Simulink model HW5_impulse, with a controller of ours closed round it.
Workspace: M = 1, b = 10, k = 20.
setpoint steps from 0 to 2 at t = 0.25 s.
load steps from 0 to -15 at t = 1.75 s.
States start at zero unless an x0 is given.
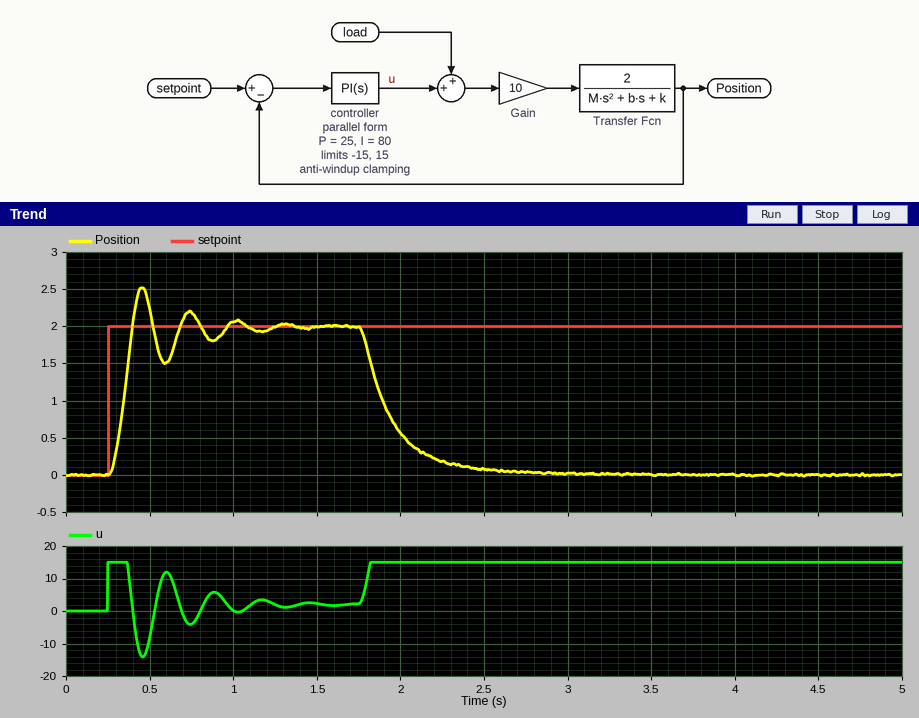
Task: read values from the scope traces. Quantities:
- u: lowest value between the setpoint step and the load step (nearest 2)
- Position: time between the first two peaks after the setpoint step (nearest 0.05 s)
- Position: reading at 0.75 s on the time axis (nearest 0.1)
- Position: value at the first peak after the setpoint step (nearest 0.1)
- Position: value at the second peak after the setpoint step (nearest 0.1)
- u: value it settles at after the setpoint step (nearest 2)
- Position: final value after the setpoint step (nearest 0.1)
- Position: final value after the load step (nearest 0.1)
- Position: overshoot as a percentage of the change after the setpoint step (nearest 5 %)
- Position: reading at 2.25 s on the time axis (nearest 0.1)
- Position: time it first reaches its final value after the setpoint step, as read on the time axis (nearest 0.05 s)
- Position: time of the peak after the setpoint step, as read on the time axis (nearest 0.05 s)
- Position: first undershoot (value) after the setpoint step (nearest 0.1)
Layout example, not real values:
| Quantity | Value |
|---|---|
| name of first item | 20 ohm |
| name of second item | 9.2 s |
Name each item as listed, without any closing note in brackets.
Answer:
| Quantity | Value |
|---|---|
| u: lowest value between the setpoint step and the load step | -14 |
| Position: time between the first two peaks after the setpoint step | 0.30 s |
| Position: reading at 0.75 s on the time axis | 2.2 |
| Position: value at the first peak after the setpoint step | 2.5 |
| Position: value at the second peak after the setpoint step | 2.2 |
| u: value it settles at after the setpoint step | 2 |
| Position: final value after the setpoint step | 2.0 |
| Position: final value after the load step | 0.0 |
| Position: overshoot as a percentage of the change after the setpoint step | 25 % |
| Position: reading at 2.25 s on the time axis | 0.2 |
| Position: time it first reaches its final value after the setpoint step, as read on the time axis | 0.40 s |
| Position: time of the peak after the setpoint step, as read on the time axis | 0.45 s |
| Position: first undershoot (value) after the setpoint step | 1.5 |
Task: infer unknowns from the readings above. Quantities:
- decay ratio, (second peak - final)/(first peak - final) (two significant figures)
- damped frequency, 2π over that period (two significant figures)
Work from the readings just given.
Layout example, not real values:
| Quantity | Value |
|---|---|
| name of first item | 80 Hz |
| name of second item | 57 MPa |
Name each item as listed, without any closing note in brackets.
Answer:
| Quantity | Value |
|---|---|
| decay ratio, (second peak - final)/(first peak - final) | 0.40 |
| damped frequency, 2π over that period | 21 rad/s |
